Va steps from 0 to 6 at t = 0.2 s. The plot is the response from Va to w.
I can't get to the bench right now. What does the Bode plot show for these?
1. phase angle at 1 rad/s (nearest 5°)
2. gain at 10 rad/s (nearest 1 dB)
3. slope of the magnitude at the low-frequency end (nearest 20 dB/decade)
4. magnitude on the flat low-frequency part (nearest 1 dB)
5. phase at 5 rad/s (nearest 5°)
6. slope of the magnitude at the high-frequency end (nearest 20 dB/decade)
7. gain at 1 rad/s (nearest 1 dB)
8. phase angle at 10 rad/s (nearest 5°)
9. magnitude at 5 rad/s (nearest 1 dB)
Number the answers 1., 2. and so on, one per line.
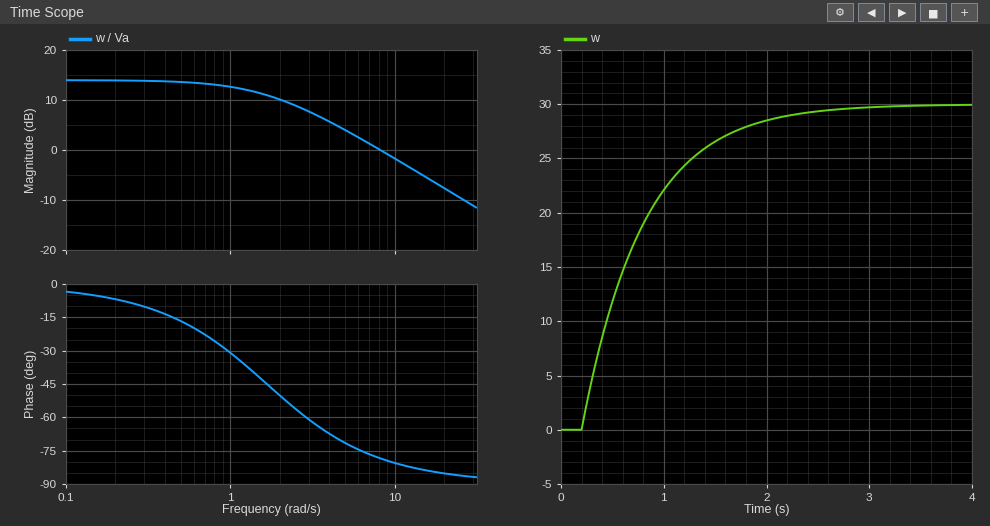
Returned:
1. -30°
2. -2 dB
3. 0 dB/decade
4. 14 dB
5. -70°
6. -20 dB/decade
7. 13 dB
8. -80°
9. 4 dB
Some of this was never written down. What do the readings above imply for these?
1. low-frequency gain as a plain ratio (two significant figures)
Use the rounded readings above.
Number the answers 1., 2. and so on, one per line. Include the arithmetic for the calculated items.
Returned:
1. 10^(14 / 20) = 5.0
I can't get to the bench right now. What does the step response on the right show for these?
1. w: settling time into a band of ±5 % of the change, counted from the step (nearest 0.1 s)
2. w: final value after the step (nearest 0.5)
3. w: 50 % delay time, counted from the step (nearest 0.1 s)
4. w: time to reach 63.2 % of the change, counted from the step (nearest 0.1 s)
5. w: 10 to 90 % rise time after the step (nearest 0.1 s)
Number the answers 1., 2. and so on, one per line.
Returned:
1. 1.8 s
2. 30.0
3. 0.4 s
4. 0.6 s
5. 1.3 s
